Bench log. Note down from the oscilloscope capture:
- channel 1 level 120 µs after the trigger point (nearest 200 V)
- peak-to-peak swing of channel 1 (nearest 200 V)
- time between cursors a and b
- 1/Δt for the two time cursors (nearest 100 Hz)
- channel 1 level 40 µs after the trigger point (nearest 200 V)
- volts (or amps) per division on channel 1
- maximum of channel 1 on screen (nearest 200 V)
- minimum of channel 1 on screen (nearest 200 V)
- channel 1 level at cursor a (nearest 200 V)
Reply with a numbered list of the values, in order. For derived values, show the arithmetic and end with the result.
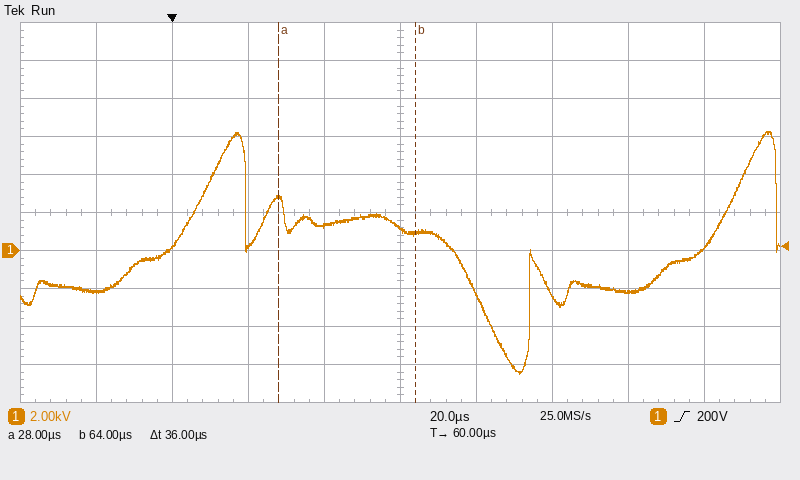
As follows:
1. -2.2 kV
2. 6.2 kV − (-6.6 kV) = 12.8 kV
3. 36 µs
4. 1 / 36 µs ≈ 27.8 kHz
5. 1.2 kV
6. 2 kV
7. 6.2 kV
8. -6.6 kV
9. 2.8 kV
